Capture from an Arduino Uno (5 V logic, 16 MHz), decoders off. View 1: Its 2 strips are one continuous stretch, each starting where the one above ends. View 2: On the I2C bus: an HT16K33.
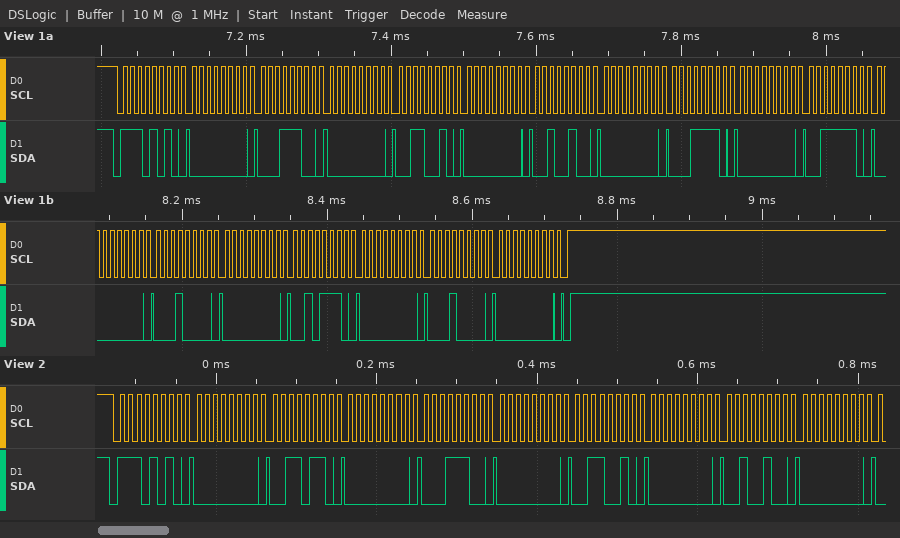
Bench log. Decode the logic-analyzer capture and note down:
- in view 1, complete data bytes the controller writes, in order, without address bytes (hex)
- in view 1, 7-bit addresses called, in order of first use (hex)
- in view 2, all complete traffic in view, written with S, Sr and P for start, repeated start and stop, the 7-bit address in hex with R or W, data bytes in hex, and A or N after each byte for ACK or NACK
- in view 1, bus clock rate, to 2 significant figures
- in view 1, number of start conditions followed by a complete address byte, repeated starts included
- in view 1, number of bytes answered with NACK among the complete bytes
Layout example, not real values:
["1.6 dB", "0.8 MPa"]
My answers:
["00 1C 00 32 00 24 00 1E 00 3E 00 10 00 2E 00 10 00", "0x75", "S 75W A 00 A 36 A 00 A 1C A 00 A 32 A 00 A 24 A 00 A", "100 kHz", "1", "0"]
